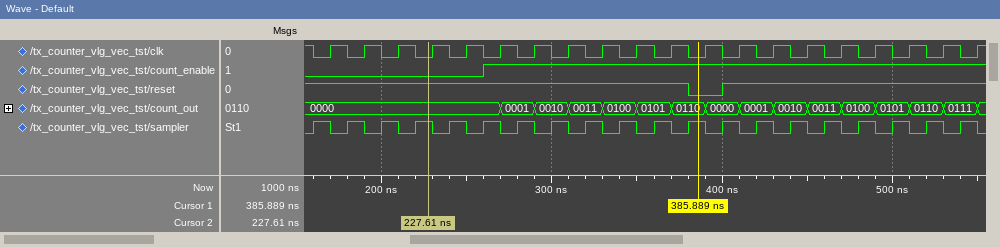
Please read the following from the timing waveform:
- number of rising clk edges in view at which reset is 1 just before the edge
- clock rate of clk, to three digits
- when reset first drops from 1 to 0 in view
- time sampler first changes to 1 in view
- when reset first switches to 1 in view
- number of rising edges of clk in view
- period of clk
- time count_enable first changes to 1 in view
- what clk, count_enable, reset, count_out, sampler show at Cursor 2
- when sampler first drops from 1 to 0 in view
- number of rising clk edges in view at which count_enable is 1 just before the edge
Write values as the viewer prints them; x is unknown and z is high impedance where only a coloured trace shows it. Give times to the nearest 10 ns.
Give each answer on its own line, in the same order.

19
50.0 MHz
380 ns
160 ns
400 ns
20
20 ns
260 ns
clk=0, count_enable=0, reset=1, count_out=0000, sampler=1
170 ns
15
